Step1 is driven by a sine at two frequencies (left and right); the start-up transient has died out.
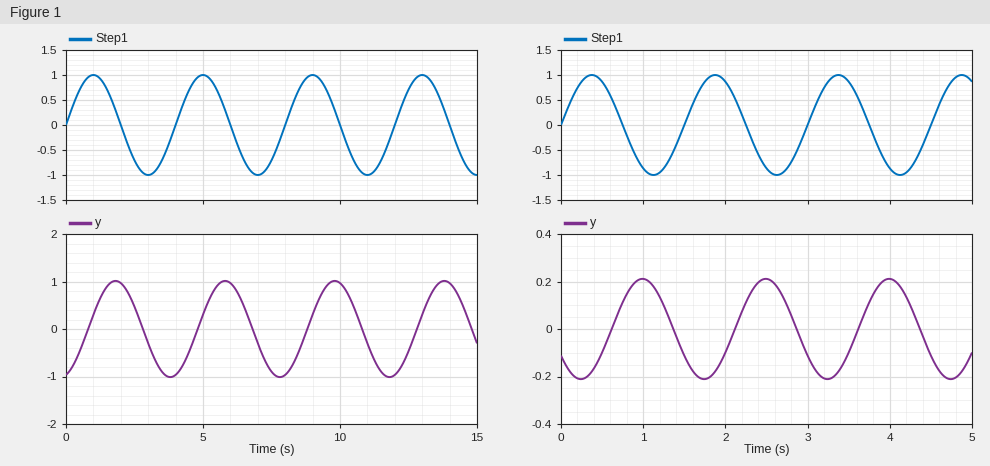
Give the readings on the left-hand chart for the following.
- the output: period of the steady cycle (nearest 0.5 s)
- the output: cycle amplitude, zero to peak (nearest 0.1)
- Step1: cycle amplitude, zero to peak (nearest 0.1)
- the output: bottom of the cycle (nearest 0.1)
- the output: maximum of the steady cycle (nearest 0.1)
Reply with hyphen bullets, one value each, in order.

- 4.0 s
- 1.0
- 1.0
- -1.0
- 1.0
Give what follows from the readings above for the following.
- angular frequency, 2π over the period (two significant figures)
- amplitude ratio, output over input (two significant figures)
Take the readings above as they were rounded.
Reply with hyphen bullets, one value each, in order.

- 1.6 rad/s
- 1.0
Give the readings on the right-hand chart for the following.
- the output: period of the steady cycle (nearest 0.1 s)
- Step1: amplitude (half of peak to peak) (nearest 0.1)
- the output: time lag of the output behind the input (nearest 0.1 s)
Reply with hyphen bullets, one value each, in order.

- 1.5 s
- 1.0
- 0.6 s
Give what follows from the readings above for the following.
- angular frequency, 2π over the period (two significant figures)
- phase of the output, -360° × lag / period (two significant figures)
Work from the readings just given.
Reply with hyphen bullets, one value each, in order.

- 4.2 rad/s
- -140°
